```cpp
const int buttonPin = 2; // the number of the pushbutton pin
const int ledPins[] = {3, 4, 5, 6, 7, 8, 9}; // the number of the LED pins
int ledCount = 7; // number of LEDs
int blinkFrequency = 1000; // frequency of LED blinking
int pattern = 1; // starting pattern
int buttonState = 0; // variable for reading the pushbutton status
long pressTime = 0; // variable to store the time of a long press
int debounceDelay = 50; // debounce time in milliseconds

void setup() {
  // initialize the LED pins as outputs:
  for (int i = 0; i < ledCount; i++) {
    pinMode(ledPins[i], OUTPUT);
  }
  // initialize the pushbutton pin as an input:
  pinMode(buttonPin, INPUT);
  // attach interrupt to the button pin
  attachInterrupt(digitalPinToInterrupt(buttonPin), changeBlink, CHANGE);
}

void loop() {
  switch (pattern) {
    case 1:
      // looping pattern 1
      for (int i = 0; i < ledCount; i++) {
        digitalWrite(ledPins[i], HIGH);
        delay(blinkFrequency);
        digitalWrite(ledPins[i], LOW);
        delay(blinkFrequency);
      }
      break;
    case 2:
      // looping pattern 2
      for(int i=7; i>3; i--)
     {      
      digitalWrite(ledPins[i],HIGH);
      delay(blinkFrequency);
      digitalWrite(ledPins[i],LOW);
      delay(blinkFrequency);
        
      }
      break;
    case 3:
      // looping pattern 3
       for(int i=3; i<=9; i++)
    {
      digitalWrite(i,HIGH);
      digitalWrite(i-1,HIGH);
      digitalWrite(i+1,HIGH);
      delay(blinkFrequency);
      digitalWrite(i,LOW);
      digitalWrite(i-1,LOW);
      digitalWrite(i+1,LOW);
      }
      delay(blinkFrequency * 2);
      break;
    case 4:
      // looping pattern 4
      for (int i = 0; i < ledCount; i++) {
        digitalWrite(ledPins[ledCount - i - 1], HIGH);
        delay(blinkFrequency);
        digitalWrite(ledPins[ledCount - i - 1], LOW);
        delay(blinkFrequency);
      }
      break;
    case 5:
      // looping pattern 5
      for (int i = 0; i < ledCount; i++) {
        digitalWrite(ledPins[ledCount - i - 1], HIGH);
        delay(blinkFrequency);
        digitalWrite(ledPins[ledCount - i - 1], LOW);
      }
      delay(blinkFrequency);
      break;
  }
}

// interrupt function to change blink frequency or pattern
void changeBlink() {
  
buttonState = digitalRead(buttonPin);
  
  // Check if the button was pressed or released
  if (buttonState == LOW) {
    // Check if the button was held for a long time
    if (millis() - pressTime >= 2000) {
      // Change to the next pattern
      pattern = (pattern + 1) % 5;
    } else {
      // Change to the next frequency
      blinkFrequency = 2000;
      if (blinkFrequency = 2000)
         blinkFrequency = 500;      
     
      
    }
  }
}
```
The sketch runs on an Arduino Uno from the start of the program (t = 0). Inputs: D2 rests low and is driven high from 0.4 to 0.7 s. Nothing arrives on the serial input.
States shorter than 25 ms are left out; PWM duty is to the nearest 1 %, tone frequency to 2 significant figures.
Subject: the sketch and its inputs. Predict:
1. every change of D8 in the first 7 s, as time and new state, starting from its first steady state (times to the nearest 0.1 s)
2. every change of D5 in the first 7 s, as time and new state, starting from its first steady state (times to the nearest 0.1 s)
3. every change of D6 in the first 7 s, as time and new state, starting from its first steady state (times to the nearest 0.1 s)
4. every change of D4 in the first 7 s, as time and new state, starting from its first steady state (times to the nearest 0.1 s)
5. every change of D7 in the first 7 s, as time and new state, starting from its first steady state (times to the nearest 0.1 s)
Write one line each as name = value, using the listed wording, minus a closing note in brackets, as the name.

every change of D8 in the first 7 s, as time and new state, starting from its first steady state = 0 s low; 5.5 s high; 6 s low
every change of D5 in the first 7 s, as time and new state, starting from its first steady state = 0 s low; 2.5 s high; 3 s low
every change of D6 in the first 7 s, as time and new state, starting from its first steady state = 0 s low; 3.5 s high; 4 s low
every change of D4 in the first 7 s, as time and new state, starting from its first steady state = 0 s low; 1.5 s high; 2 s low
every change of D7 in the first 7 s, as time and new state, starting from its first steady state = 0 s low; 4.5 s high; 5 s low
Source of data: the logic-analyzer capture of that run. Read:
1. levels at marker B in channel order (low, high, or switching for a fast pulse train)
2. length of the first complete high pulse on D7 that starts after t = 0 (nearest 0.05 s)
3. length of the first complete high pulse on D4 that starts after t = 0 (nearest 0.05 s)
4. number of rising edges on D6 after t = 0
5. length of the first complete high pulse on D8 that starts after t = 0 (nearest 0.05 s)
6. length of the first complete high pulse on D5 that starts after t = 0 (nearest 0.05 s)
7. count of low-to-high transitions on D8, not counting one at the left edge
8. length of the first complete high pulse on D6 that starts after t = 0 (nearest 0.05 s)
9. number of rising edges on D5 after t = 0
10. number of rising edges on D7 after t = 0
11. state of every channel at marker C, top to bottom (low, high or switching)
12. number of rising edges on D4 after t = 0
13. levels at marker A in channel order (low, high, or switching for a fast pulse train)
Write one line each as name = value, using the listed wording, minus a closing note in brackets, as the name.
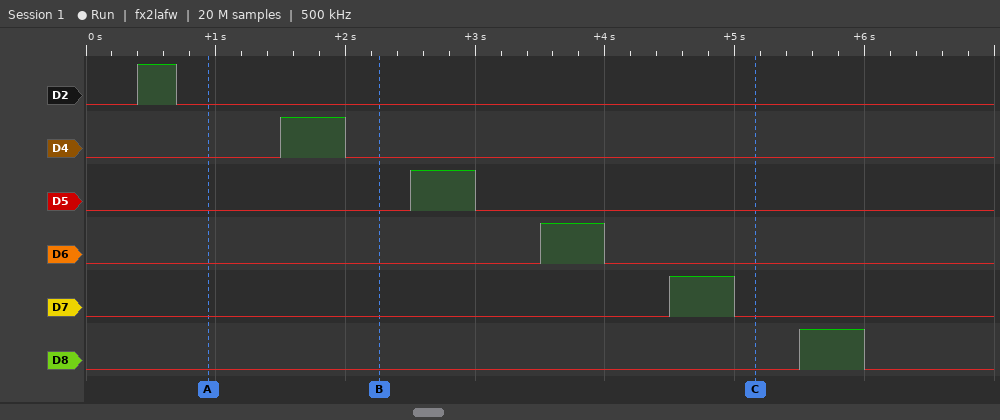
levels at marker B in channel order = D2 low, D4 low, D5 low, D6 low, D7 low, D8 low
length of the first complete high pulse on D7 that starts after t = 0 = 0.50 s
length of the first complete high pulse on D4 that starts after t = 0 = 0.50 s
number of rising edges on D6 after t = 0 = 1
length of the first complete high pulse on D8 that starts after t = 0 = 0.50 s
length of the first complete high pulse on D5 that starts after t = 0 = 0.50 s
count of low-to-high transitions on D8, not counting one at the left edge = 1
length of the first complete high pulse on D6 that starts after t = 0 = 0.50 s
number of rising edges on D5 after t = 0 = 1
number of rising edges on D7 after t = 0 = 1
state of every channel at marker C, top to bottom = D2 low, D4 low, D5 low, D6 low, D7 low, D8 low
number of rising edges on D4 after t = 0 = 1
levels at marker A in channel order = D2 low, D4 low, D5 low, D6 low, D7 low, D8 low
